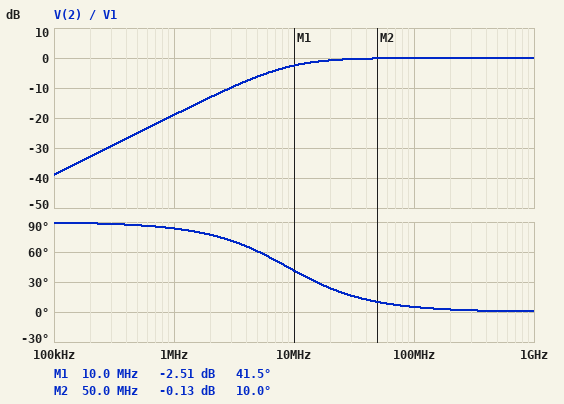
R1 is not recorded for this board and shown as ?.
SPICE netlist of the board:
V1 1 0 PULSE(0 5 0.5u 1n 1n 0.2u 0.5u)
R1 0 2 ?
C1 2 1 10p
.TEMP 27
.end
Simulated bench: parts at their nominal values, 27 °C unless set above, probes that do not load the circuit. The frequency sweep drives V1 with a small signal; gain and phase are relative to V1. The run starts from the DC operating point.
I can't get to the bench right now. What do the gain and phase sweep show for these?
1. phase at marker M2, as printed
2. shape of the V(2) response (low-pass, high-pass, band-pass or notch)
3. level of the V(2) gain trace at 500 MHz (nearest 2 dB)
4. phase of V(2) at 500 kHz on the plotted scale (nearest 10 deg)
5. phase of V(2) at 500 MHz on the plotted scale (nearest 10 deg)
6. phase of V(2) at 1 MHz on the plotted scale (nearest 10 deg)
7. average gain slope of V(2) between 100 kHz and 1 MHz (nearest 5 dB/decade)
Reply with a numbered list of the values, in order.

1. 10.0 deg
2. high-pass
3. 0 dB
4. 90 deg
5. 0 deg
6. 80 deg
7. 20 dB/decade
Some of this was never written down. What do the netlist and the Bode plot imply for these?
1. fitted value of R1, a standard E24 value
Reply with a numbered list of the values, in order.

1. 1.8 kΩ
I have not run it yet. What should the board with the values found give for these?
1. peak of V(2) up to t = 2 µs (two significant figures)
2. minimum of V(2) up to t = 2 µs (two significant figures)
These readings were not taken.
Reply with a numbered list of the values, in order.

1. 4.9 V
2. -4.9 V
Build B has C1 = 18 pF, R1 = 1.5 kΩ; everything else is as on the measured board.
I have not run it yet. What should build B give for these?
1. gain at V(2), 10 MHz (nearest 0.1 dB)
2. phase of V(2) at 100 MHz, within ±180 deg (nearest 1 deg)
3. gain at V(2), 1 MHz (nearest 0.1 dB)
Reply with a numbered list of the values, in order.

1. -1.3 dB
2. 3 deg
3. -15.5 dB
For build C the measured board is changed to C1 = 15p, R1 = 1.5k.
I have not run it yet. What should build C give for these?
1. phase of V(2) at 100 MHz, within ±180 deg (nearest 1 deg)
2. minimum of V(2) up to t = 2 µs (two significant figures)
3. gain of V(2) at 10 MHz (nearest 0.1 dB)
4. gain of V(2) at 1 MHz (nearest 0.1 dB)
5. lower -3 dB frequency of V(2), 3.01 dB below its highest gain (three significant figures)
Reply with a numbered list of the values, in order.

1. 4 deg
2. -4.9 V
3. -1.8 dB
4. -17.1 dB
5. 7.07 MHz
